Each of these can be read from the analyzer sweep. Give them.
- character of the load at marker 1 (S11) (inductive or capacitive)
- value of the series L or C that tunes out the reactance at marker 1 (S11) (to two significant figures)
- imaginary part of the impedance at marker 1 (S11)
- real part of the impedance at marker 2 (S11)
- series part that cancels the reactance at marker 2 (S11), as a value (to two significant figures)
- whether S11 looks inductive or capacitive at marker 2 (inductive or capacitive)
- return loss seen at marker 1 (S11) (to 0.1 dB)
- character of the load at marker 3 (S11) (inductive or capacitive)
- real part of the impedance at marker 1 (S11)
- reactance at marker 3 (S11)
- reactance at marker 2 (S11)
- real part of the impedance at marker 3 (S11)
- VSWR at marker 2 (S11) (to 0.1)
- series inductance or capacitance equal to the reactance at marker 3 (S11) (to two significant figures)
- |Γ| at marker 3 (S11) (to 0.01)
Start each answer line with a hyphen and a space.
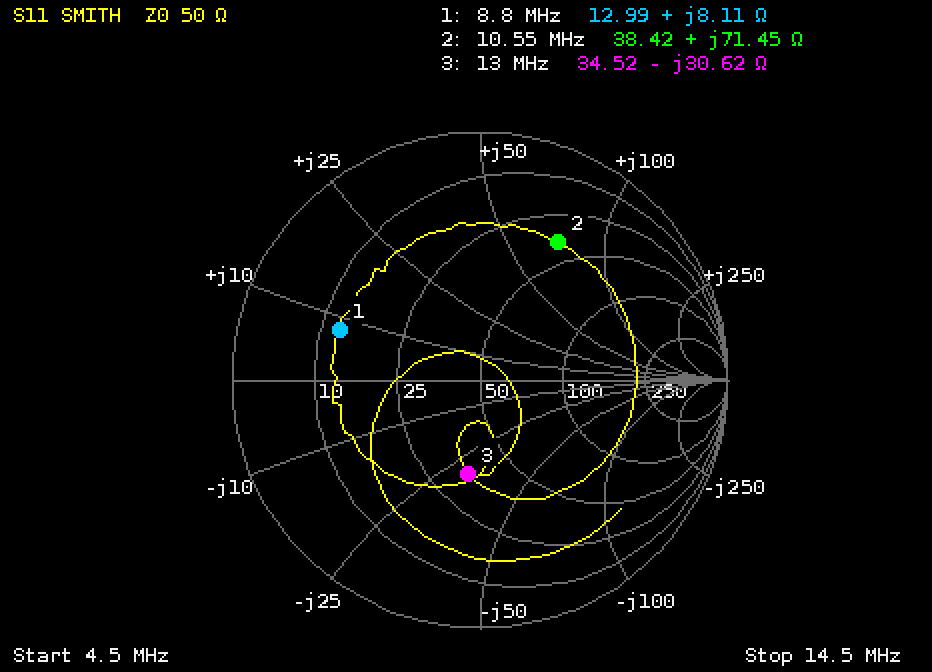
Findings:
- inductive
- 2.2 nF
- +8.11 Ω
- 38.42 Ω
- 210 pF
- inductive
- 4.5 dB
- capacitive
- 12.99 Ω
- -30.62 Ω
- +71.45 Ω
- 34.52 Ω
- 4.5
- 400 pF
- 0.38
